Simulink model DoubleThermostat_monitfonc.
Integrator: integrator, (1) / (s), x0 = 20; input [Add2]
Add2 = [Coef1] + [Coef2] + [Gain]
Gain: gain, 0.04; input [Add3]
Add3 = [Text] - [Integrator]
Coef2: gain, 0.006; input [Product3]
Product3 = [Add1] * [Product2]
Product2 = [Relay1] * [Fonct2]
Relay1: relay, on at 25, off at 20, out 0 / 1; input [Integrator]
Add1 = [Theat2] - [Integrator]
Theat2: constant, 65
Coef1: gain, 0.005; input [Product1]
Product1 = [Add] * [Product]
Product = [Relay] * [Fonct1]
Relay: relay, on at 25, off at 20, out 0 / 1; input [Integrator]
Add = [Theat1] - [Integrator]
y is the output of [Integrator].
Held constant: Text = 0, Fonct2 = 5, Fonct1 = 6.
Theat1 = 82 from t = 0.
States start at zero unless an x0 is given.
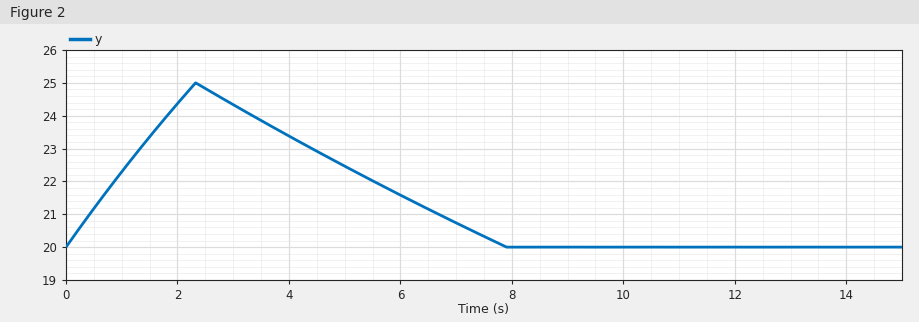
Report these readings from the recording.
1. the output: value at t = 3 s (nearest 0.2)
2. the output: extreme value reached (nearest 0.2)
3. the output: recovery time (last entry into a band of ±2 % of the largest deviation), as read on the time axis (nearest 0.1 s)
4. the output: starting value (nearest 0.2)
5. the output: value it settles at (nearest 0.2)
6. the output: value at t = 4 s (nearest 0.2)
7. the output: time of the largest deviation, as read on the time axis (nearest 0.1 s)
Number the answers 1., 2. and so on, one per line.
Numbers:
1. 24.4
2. 25.0
3. 7.8 s
4. 20.0
5. 20.0
6. 23.4
7. 2.3 s
